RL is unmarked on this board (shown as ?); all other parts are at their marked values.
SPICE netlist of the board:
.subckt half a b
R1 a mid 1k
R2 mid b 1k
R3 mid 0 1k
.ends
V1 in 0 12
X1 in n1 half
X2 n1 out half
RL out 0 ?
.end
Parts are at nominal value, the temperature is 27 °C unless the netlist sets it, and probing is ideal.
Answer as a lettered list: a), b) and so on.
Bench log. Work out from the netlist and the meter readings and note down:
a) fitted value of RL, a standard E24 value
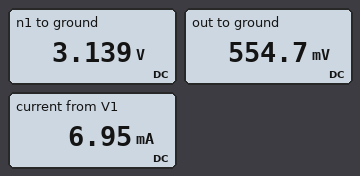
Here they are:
a) 820 Ω
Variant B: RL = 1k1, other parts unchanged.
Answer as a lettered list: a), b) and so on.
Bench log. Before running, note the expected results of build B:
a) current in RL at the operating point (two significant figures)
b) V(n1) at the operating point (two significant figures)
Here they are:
a) 610 µA
b) 3.2 V
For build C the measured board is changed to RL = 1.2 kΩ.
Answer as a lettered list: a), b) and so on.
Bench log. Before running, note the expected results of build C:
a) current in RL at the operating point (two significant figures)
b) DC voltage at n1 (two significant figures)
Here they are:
a) 590 µA
b) 3.2 V
